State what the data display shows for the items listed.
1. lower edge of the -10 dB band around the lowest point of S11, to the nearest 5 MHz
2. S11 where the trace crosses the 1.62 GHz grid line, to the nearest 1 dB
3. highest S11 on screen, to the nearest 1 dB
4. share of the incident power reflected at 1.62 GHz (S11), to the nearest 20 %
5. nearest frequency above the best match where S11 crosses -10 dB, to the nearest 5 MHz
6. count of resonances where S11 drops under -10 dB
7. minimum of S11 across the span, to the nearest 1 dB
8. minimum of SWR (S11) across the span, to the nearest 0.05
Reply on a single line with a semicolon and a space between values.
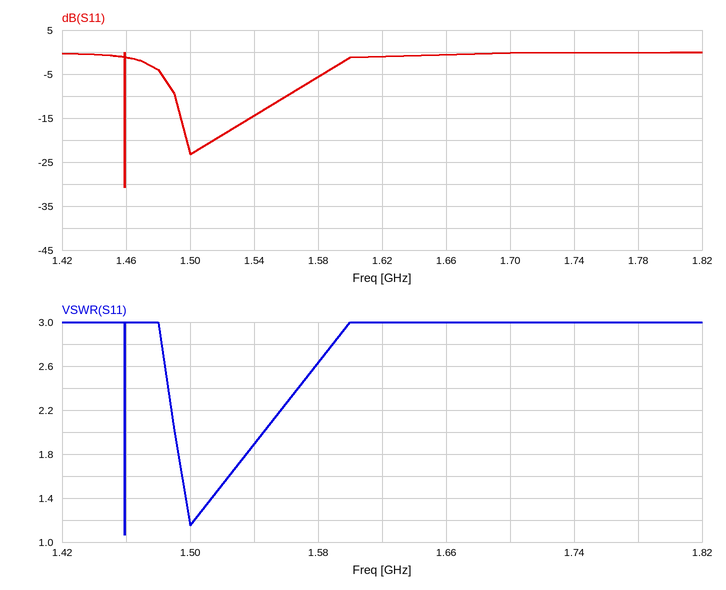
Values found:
1.460 GHz; -1 dB; 0 dB; 80 %; 1.460 GHz; 2; -31 dB; 1.05
